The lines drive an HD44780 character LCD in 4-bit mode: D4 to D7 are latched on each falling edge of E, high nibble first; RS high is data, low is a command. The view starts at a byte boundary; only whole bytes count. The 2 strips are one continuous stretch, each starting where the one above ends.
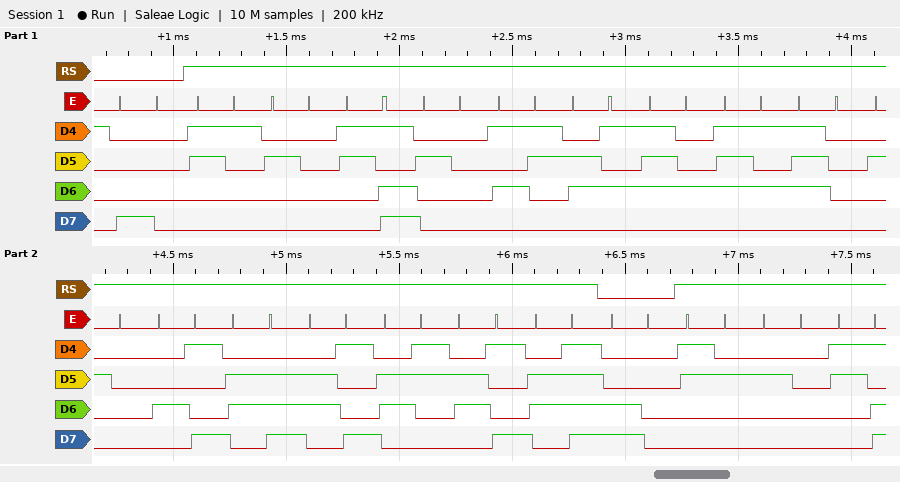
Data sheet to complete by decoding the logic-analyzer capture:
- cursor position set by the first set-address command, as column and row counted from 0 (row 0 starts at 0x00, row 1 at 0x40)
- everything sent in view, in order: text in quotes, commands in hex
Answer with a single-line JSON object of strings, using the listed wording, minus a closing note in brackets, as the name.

{"cursor position set by the first set-address command, as column and row counted from 0": "column 0, row 0", "everything sent in view, in order: text in quotes, commands in hex": "0x80 \"1 = Setup Inicio\" 0xC0 \"2 =\""}
